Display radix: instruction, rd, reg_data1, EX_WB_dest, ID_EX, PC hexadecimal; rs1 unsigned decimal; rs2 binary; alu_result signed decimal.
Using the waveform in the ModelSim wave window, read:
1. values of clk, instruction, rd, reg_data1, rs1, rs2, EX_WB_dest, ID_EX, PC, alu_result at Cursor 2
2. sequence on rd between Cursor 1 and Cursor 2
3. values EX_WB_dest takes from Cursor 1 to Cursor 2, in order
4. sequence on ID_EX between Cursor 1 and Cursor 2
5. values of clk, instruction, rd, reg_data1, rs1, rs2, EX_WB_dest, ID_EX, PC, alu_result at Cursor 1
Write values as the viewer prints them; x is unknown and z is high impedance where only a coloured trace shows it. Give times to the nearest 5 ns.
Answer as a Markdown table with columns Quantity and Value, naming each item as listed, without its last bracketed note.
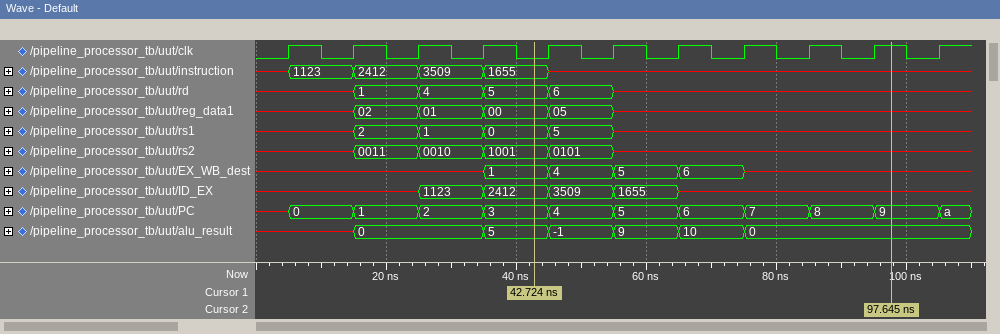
| Quantity | Value |
|---|---|
| values of clk, instruction, rd, reg_data1, rs1, rs2, EX_WB_dest, ID_EX, PC, alu_result at Cursor 2 | clk=1, instruction=x, rd=x, reg_data1=x, rs1=x, rs2=x, EX_WB_dest=x, ID_EX=x, PC=9, alu_result=0 |
| sequence on rd between Cursor 1 and Cursor 2 | 5, 6, x |
| values EX_WB_dest takes from Cursor 1 to Cursor 2, in order | 1, 4, 5, 6, x |
| sequence on ID_EX between Cursor 1 and Cursor 2 | 2412, 3509, 1655, x |
| values of clk, instruction, rd, reg_data1, rs1, rs2, EX_WB_dest, ID_EX, PC, alu_result at Cursor 1 | clk=0, instruction=1655, rd=5, reg_data1=00, rs1=0, rs2=1001, EX_WB_dest=1, ID_EX=2412, PC=3, alu_result=5 |
